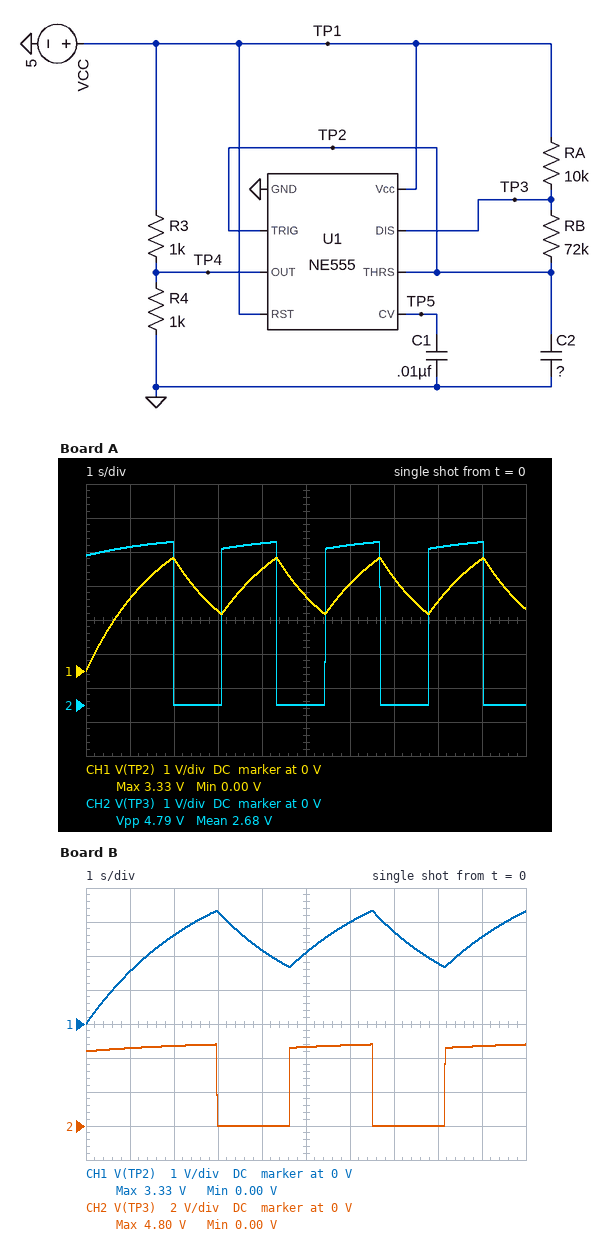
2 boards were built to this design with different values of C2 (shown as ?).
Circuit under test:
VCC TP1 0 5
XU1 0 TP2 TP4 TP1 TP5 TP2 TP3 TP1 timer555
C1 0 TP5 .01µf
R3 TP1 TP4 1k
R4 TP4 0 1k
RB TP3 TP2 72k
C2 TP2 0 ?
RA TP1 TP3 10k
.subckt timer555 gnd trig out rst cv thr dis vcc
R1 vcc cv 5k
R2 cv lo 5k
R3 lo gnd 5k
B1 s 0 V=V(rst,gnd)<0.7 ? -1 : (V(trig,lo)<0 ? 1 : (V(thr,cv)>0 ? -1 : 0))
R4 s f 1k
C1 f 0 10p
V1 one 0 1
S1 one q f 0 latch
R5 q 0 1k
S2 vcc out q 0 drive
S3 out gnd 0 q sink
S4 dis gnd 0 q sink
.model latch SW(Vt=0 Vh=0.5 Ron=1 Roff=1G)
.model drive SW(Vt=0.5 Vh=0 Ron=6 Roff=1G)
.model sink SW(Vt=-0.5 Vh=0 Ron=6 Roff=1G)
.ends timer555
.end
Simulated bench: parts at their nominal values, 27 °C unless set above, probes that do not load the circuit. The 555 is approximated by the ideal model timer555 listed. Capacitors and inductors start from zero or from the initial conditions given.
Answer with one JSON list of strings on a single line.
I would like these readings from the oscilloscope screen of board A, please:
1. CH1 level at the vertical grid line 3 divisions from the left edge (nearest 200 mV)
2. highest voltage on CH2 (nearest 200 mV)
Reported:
["1.8 V", "4.8 V"]
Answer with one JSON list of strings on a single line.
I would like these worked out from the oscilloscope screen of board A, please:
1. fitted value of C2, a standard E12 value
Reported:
["22 µF"]
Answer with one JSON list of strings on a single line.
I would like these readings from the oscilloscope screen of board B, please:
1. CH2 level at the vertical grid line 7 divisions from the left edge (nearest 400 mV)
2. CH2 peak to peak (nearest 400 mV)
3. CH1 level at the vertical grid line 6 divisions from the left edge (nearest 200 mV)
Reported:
["0 V", "4.8 V", "3.0 V"]
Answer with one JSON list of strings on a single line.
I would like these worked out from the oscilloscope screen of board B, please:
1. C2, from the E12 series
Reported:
["33 µF"]
